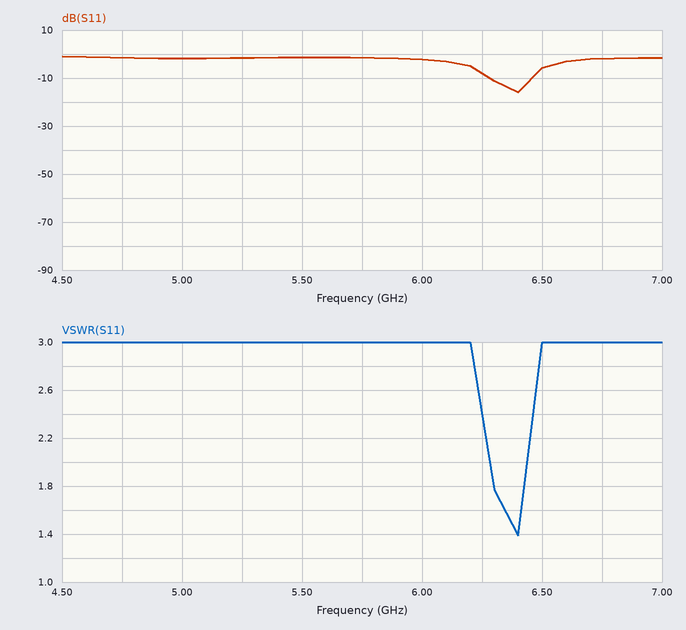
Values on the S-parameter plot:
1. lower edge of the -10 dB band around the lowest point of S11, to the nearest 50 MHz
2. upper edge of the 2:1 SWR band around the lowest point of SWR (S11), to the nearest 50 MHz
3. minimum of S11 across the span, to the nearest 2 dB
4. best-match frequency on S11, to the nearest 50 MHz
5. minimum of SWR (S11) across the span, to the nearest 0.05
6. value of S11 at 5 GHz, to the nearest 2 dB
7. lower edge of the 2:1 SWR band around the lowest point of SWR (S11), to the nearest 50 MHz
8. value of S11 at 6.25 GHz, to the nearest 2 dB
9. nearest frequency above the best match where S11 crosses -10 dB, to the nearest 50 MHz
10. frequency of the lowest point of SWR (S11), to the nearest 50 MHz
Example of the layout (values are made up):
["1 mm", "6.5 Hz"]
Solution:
["6.30 GHz", "6.45 GHz", "-16 dB", "6.40 GHz", "1.40", "-2 dB", "6.30 GHz", "-8 dB", "6.45 GHz", "6.40 GHz"]
